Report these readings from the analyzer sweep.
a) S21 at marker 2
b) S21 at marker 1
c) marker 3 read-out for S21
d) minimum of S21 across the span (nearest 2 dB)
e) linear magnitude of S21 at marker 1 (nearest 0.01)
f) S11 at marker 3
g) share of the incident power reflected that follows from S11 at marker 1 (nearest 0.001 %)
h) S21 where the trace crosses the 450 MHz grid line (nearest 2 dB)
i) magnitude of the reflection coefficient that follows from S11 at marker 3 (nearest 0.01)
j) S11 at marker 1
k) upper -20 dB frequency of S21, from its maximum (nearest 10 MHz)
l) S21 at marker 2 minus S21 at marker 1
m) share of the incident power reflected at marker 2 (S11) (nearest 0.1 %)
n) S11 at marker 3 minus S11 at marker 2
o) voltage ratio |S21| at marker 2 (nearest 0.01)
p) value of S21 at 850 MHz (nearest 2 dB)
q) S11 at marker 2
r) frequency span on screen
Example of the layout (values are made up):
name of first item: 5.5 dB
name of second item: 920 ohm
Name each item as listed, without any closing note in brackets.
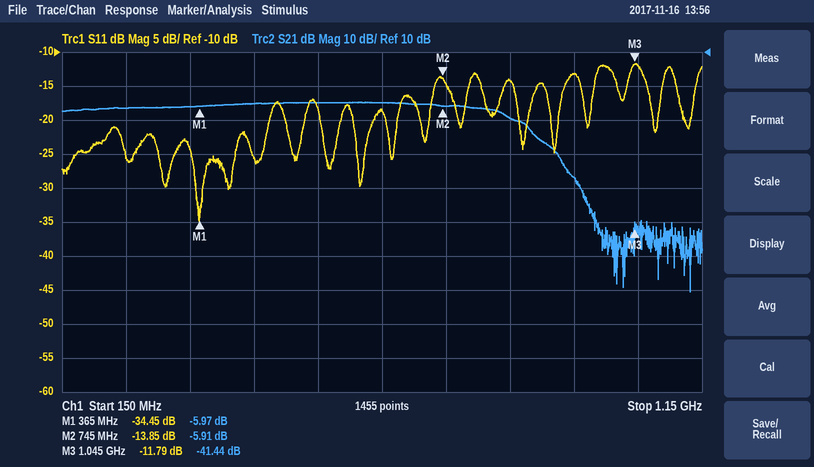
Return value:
S21 at marker 2: -5.91 dB
S21 at marker 1: -5.97 dB
marker 3 read-out for S21: -41.44 dB
minimum of S21 across the span: -60 dB
linear magnitude of S21 at marker 1: 0.50
S11 at marker 3: -11.79 dB
share of the incident power reflected that follows from S11 at marker 1: 0.036 %
S21 where the trace crosses the 450 MHz grid line: -6 dB
magnitude of the reflection coefficient that follows from S11 at marker 3: 0.26
S11 at marker 1: -34.45 dB
upper -20 dB frequency of S21, from its maximum: 940 MHz
S21 at marker 2 minus S21 at marker 1: 0.06 dB
share of the incident power reflected at marker 2 (S11): 4.1 %
S11 at marker 3 minus S11 at marker 2: 2.06 dB
voltage ratio |S21| at marker 2: 0.51
value of S21 at 850 MHz: -10 dB
S11 at marker 2: -13.85 dB
frequency span on screen: 1 GHz
